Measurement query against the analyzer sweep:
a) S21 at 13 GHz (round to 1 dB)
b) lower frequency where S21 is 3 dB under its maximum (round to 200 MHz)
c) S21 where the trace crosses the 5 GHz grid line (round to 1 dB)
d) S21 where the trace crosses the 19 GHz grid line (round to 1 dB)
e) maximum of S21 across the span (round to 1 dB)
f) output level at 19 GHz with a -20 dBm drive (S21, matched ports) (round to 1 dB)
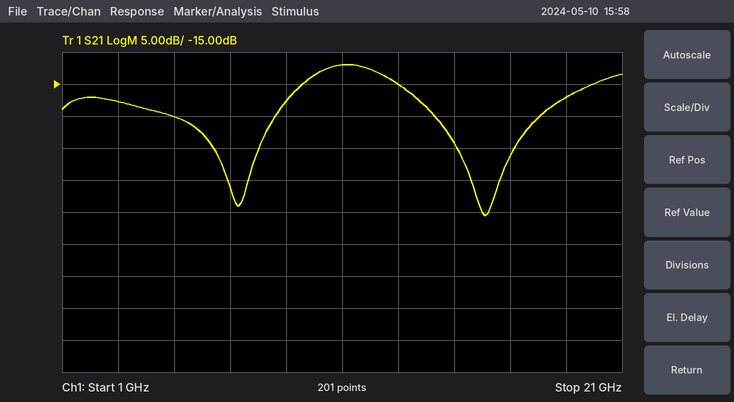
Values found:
-15 dB
9.6 GHz
-20 dB
-17 dB
-12 dB
-37 dBm
